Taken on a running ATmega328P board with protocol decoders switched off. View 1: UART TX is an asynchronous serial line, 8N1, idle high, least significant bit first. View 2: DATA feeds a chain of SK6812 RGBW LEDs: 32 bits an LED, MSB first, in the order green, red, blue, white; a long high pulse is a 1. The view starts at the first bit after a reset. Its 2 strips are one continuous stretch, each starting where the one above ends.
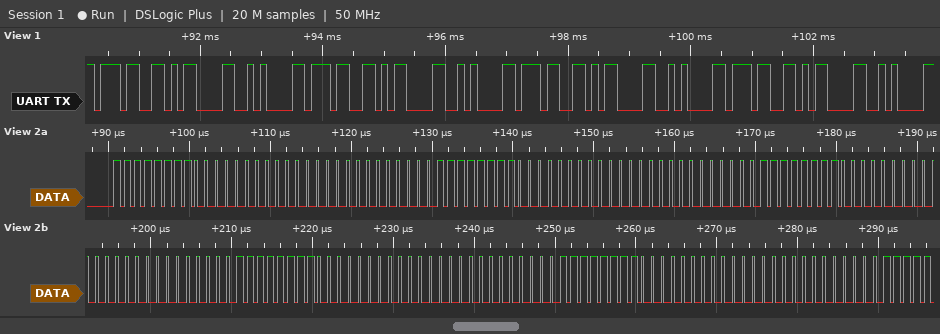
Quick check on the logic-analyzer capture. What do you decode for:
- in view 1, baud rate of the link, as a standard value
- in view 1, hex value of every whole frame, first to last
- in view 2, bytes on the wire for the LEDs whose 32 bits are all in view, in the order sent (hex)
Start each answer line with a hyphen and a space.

- 9600 baud
- 37 0D 0A 37 0D 0A 37 0D 0A 37 0D 0A
- FF 00 00 00 FF 00 00 00 FF 00 00 00 FF 00 00 00 FF 00 00 00
